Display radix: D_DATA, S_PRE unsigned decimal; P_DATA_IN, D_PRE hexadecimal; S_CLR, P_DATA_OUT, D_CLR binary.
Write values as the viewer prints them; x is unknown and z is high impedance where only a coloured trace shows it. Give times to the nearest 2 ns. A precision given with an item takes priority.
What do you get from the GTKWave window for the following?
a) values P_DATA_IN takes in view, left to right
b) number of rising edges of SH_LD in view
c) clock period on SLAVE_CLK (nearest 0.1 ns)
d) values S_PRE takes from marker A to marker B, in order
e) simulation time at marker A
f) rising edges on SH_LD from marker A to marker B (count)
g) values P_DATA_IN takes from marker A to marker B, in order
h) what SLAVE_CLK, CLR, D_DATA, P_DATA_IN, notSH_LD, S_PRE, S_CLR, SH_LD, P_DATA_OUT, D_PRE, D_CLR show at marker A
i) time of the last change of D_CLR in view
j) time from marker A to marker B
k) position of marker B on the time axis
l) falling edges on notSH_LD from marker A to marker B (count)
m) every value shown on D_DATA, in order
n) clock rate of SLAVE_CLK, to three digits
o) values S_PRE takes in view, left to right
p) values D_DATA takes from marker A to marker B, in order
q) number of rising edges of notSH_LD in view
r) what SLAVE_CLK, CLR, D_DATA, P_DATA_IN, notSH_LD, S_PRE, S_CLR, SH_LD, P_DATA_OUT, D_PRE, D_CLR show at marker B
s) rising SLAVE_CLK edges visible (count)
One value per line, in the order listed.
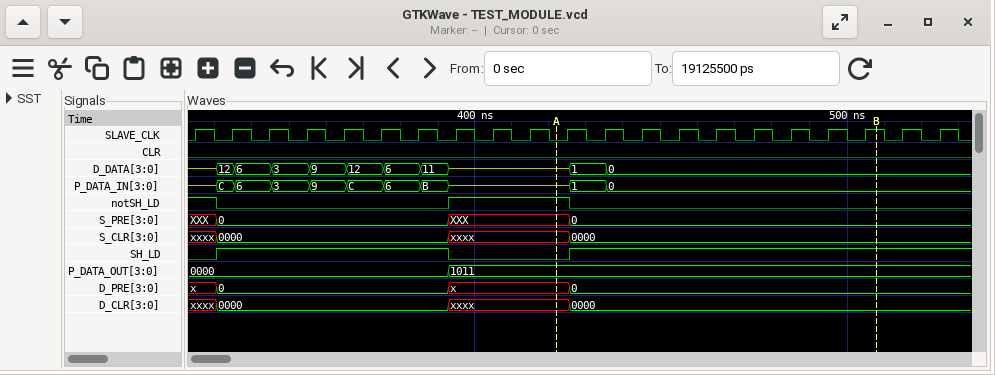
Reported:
z, C, 6, 3, 9, C, 6, B, z, 1, 0
2
10 ns
XXX, 0
422 ns
1
z, 1, 0
SLAVE_CLK=0, CLR=0, D_DATA=z, P_DATA_IN=z, notSH_LD=1, S_PRE=XXX, S_CLR=xxxx, SH_LD=0, P_DATA_OUT=1011, D_PRE=x, D_CLR=xxxx
426 ns
86 ns
508 ns
1
z, 12, 6, 3, 9, 12, 6, 11, z, 1, 0
100 MHz
XXX, 0, XXX, 0
z, 1, 0
1
SLAVE_CLK=1, CLR=0, D_DATA=0, P_DATA_IN=0, notSH_LD=0, S_PRE=0, S_CLR=0000, SH_LD=1, P_DATA_OUT=1011, D_PRE=0, D_CLR=0000
21
